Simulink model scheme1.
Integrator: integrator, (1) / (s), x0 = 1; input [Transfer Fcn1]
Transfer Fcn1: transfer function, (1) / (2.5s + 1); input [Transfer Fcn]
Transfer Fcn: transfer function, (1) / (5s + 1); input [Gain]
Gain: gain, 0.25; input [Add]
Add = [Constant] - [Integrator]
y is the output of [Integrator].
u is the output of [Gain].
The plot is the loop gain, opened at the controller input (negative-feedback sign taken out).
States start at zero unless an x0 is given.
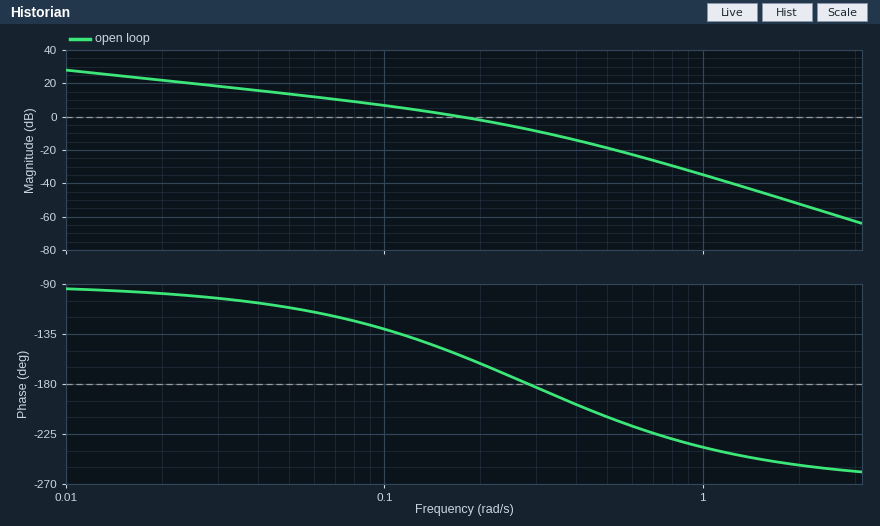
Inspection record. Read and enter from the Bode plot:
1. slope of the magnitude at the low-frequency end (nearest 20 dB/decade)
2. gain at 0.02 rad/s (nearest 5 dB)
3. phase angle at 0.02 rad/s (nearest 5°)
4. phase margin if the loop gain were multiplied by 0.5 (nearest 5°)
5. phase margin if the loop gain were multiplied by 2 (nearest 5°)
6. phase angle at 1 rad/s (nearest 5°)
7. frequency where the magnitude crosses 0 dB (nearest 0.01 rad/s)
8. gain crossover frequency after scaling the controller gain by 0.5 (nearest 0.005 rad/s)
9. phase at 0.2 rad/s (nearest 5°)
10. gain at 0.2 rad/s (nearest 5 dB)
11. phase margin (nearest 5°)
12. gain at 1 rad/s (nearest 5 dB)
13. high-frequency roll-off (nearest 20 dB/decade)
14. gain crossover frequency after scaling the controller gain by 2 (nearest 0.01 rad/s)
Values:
-20 dB/decade
20 dB
-100°
45°
5°
-235°
0.17 rad/s
0.105 rad/s
-160°
0 dB
25°
-35 dB
-60 dB/decade
0.26 rad/s
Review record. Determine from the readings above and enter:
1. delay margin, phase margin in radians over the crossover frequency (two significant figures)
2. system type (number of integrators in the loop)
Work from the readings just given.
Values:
2.6 s
1
